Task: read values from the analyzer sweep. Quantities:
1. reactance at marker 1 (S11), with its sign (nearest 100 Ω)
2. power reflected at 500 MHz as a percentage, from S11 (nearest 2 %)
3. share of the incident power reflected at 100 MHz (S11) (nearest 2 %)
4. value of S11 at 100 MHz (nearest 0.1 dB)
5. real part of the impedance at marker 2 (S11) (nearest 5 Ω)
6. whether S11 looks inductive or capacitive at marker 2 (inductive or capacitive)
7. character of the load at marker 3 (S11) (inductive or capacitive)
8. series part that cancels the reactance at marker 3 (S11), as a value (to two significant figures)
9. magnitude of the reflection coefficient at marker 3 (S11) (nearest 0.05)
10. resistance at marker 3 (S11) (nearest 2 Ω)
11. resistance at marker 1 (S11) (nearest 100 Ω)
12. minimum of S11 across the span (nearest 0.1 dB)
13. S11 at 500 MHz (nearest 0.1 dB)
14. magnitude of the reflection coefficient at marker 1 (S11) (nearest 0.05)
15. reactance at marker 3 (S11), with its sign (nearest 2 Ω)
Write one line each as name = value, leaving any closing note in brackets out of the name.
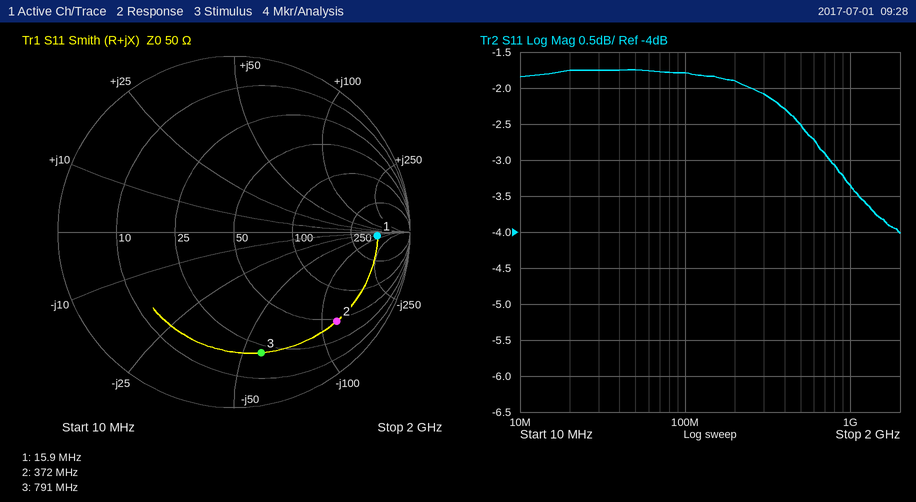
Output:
reactance at marker 1 (S11), with its sign = -100 Ω
power reflected at 500 MHz as a percentage, from S11 = 56 %
share of the incident power reflected at 100 MHz (S11) = 66 %
value of S11 at 100 MHz = -1.8 dB
real part of the impedance at marker 2 (S11) = 45 Ω
whether S11 looks inductive or capacitive at marker 2 = capacitive
character of the load at marker 3 (S11) = capacitive
series part that cancels the reactance at marker 3 (S11), as a value = 12 nH
magnitude of the reflection coefficient at marker 3 (S11) = 0.70
resistance at marker 3 (S11) = 22 Ω
resistance at marker 1 (S11) = 500 Ω
minimum of S11 across the span = -4.0 dB
S11 at 500 MHz = -2.5 dB
magnitude of the reflection coefficient at marker 1 (S11) = 0.80
reactance at marker 3 (S11), with its sign = -58 Ω
